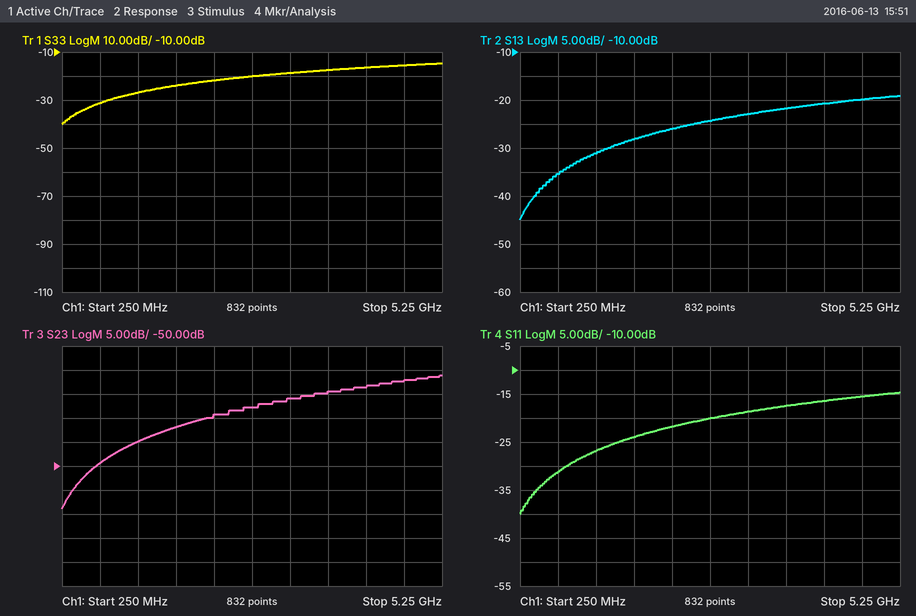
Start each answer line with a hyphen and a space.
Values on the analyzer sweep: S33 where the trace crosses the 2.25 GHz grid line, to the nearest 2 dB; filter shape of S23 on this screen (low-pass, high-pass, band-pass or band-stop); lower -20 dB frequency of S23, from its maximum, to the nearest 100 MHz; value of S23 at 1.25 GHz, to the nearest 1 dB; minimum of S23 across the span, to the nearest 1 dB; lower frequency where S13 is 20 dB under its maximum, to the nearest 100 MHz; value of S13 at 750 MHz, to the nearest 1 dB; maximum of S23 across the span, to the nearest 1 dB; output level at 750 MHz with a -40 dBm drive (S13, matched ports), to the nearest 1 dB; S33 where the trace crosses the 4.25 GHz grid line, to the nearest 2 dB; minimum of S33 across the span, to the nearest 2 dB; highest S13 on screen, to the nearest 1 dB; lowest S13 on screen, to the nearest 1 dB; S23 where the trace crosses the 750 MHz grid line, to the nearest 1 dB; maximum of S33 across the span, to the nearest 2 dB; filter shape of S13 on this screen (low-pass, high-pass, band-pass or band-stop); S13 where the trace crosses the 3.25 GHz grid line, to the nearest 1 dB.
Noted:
- -22 dB
- high-pass
- 600 MHz
- -45 dB
- -59 dB
- 500 MHz
- -35 dB
- -31 dB
- -75 dBm
- -16 dB
- -40 dB
- -19 dB
- -45 dB
- -49 dB
- -14 dB
- high-pass
- -23 dB
